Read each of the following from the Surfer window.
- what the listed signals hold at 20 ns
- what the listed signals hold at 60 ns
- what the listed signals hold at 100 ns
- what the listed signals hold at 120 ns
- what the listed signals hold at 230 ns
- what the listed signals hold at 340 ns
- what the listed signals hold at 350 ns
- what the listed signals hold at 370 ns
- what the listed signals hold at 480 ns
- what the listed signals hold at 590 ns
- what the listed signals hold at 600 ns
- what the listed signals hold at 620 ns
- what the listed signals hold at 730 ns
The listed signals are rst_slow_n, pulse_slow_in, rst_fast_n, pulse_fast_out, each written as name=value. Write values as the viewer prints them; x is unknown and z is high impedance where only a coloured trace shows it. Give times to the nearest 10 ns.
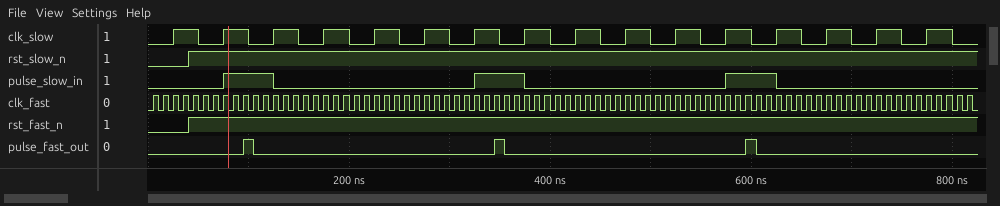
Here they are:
rst_slow_n=0, pulse_slow_in=0, rst_fast_n=0, pulse_fast_out=0
rst_slow_n=1, pulse_slow_in=0, rst_fast_n=1, pulse_fast_out=0
rst_slow_n=1, pulse_slow_in=1, rst_fast_n=1, pulse_fast_out=1
rst_slow_n=1, pulse_slow_in=1, rst_fast_n=1, pulse_fast_out=0
rst_slow_n=1, pulse_slow_in=0, rst_fast_n=1, pulse_fast_out=0
rst_slow_n=1, pulse_slow_in=1, rst_fast_n=1, pulse_fast_out=0
rst_slow_n=1, pulse_slow_in=1, rst_fast_n=1, pulse_fast_out=1
rst_slow_n=1, pulse_slow_in=1, rst_fast_n=1, pulse_fast_out=0
rst_slow_n=1, pulse_slow_in=0, rst_fast_n=1, pulse_fast_out=0
rst_slow_n=1, pulse_slow_in=1, rst_fast_n=1, pulse_fast_out=0
rst_slow_n=1, pulse_slow_in=1, rst_fast_n=1, pulse_fast_out=1
rst_slow_n=1, pulse_slow_in=1, rst_fast_n=1, pulse_fast_out=0
rst_slow_n=1, pulse_slow_in=0, rst_fast_n=1, pulse_fast_out=0
